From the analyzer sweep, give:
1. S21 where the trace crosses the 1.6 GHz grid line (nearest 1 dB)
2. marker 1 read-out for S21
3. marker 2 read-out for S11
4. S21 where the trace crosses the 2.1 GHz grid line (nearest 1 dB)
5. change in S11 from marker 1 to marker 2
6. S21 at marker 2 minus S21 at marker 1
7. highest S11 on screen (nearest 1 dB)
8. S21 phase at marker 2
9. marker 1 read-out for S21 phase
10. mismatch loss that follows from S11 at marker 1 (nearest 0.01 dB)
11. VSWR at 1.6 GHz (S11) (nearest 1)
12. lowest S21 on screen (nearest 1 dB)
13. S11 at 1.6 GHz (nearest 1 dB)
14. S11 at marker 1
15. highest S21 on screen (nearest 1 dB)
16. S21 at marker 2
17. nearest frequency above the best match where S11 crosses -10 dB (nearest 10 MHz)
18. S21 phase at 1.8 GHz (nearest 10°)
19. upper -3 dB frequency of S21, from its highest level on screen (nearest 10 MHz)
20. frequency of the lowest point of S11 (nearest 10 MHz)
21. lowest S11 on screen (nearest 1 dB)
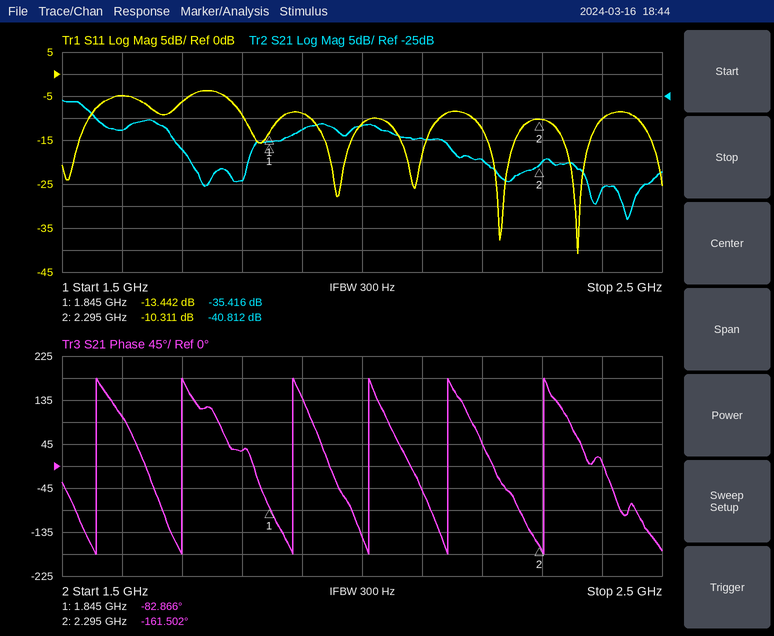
-33 dB
-35.416 dB
-10.311 dB
-35 dB
3.131 dB
-5.396 dB
-4 dB
-161.502°
-82.866°
0.20 dB
4
-53 dB
-5 dB
-13.442 dB
-26 dB
-40.812 dB
2.40 GHz
30°
1.55 GHz
2.36 GHz
-41 dB
